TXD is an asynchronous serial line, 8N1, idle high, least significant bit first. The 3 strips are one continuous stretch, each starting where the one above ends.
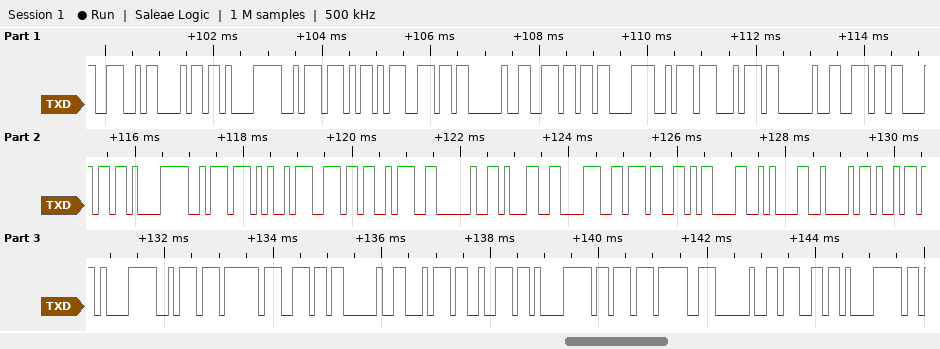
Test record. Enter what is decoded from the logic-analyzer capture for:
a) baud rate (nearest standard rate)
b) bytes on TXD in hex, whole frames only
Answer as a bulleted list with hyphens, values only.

- 9600 baud
- 4E 68 E1 BA AD 6E 20 6E C3 BA 74 20 6E 68 E1 BA A5 6E 3A 20 31 38 37 0D 0A 42 69 E1 BA BF 6E 20 74 72 E1 BB 9F 20 67 E1
